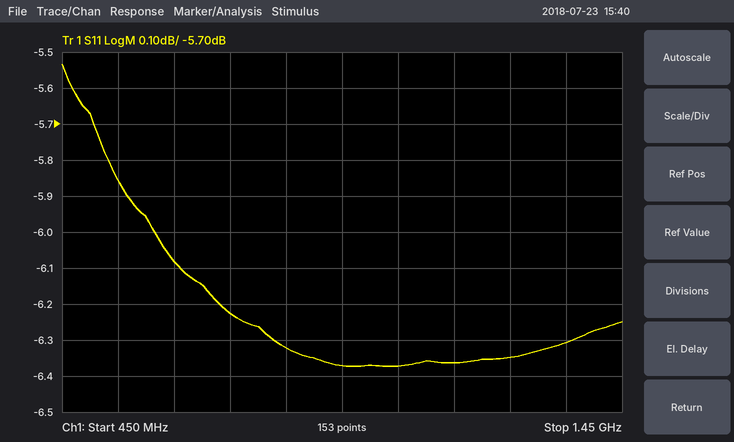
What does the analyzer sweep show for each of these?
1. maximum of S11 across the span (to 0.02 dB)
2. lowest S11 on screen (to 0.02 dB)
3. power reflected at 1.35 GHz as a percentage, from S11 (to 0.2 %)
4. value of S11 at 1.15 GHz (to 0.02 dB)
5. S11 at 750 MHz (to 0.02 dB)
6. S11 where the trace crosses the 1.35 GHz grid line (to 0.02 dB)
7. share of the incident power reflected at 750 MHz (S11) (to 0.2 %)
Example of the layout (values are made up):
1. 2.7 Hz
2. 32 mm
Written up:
1. -5.54 dB
2. -6.38 dB
3. 23.4 %
4. -6.36 dB
5. -6.22 dB
6. -6.30 dB
7. 23.8 %
